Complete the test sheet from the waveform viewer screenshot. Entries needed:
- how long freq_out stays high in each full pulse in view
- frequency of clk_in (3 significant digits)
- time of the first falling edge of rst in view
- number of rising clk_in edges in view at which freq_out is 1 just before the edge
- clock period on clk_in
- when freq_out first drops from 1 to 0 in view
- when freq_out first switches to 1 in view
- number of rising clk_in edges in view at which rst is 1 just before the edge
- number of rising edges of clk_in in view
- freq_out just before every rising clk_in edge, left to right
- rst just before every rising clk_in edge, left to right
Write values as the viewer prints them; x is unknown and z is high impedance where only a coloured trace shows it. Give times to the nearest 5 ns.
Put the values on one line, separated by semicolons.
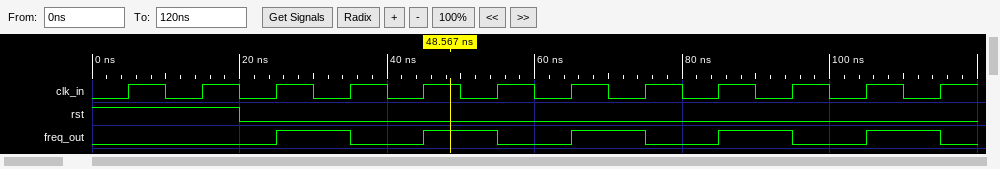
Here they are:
10 ns, 10 ns, 10 ns, 10 ns, 10 ns; 100 MHz; 20 ns; 5; 10 ns; 35 ns; 25 ns; 2; 12; 0 0 0 1 0 1 0 1 0 1 0 1; 1 1 0 0 0 0 0 0 0 0 0 0
